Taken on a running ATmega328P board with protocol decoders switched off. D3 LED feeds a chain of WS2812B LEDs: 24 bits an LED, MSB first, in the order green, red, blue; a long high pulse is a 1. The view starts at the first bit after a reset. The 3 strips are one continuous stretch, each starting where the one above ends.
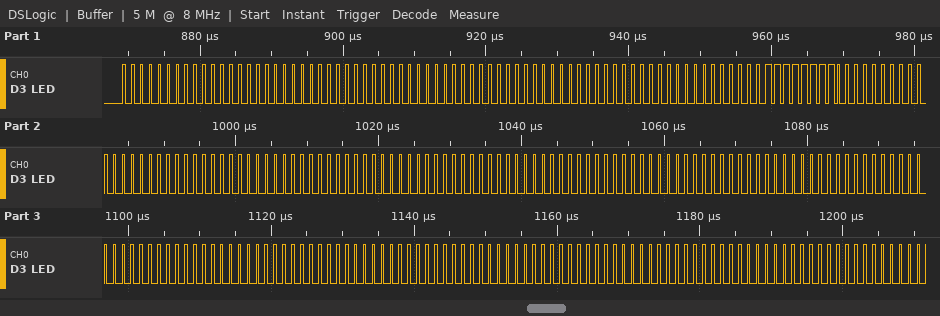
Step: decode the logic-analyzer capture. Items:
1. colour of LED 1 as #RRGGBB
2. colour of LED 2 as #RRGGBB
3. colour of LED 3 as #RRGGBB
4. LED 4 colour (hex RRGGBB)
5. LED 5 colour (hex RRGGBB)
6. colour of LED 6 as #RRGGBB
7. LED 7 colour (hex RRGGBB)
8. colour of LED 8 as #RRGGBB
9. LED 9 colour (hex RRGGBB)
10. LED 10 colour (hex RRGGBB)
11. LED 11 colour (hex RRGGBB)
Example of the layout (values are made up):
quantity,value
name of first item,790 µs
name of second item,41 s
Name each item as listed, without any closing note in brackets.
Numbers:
quantity,value
colour of LED 1 as #RRGGBB,#000000
colour of LED 2 as #RRGGBB,#000000
colour of LED 3 as #RRGGBB,#000000
LED 4 colour,#00FF00
LED 5 colour,#000000
colour of LED 6 as #RRGGBB,#000000
LED 7 colour,#000000
colour of LED 8 as #RRGGBB,#000000
LED 9 colour,#000000
LED 10 colour,#000000
LED 11 colour,#000000
